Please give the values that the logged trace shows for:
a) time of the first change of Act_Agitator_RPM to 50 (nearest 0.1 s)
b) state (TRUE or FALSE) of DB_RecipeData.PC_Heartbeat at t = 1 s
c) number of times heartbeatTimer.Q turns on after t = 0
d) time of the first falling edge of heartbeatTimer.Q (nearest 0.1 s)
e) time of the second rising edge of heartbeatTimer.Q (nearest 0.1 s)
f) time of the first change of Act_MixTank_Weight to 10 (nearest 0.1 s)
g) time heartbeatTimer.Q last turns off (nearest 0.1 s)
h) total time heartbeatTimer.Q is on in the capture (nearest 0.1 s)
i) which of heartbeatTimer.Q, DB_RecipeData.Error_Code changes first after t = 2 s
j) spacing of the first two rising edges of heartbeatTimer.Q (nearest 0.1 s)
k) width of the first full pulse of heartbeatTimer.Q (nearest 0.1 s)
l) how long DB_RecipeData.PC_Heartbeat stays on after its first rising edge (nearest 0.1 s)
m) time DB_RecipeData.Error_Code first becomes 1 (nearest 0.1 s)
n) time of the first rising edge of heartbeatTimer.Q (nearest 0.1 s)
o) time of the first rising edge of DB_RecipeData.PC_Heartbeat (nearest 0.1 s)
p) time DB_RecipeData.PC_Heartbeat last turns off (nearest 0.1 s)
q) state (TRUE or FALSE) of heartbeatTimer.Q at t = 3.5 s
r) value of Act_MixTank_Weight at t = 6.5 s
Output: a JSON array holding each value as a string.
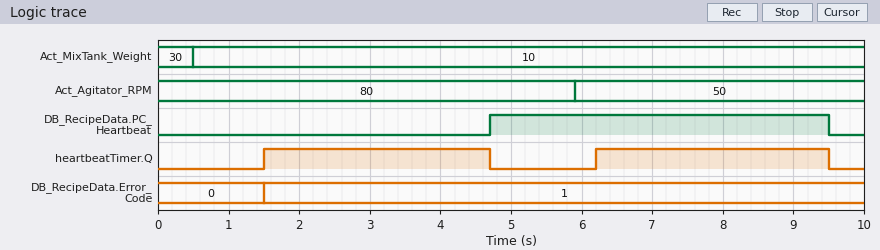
["5.9 s", "FALSE", "2", "4.7 s", "6.2 s", "0.5 s", "9.5 s", "6.5 s", "heartbeatTimer.Q", "4.7 s", "3.2 s", "4.8 s", "1.5 s", "1.5 s", "4.7 s", "9.5 s", "TRUE", "10"]
